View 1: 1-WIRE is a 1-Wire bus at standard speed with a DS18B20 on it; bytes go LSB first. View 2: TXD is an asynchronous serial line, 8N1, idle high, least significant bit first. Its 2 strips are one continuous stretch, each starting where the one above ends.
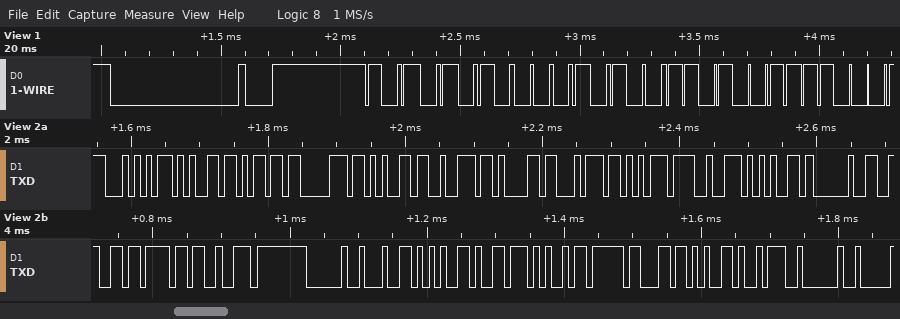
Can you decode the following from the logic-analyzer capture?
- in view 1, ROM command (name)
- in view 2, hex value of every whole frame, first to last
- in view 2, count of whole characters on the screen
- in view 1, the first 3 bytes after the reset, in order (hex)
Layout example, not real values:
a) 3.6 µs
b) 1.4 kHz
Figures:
a) Match ROM
b) 54 65 6D 70 65 72 61 74 75 72 65 20 66 6F 72 20 64 65 76 69 63 65 3A 20
c) 24
d) 55 28 CB
